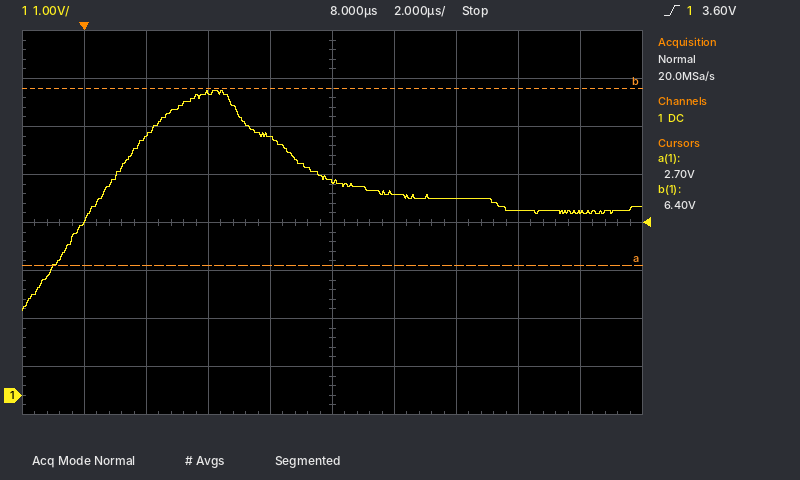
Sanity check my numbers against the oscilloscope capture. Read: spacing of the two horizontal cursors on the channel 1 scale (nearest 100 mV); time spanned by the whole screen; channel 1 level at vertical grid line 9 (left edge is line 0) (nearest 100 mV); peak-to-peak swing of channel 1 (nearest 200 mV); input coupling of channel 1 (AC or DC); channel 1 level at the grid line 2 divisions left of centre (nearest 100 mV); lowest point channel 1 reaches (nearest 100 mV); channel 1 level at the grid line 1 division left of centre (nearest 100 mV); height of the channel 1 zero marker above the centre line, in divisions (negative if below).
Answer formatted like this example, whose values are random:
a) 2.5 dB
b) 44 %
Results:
a) 3.7 V
b) 20 µs
c) 3.8 V
d) 4.6 V
e) DC
f) 6.3 V
g) 1.8 V
h) 5.4 V
i) -3.6 div
